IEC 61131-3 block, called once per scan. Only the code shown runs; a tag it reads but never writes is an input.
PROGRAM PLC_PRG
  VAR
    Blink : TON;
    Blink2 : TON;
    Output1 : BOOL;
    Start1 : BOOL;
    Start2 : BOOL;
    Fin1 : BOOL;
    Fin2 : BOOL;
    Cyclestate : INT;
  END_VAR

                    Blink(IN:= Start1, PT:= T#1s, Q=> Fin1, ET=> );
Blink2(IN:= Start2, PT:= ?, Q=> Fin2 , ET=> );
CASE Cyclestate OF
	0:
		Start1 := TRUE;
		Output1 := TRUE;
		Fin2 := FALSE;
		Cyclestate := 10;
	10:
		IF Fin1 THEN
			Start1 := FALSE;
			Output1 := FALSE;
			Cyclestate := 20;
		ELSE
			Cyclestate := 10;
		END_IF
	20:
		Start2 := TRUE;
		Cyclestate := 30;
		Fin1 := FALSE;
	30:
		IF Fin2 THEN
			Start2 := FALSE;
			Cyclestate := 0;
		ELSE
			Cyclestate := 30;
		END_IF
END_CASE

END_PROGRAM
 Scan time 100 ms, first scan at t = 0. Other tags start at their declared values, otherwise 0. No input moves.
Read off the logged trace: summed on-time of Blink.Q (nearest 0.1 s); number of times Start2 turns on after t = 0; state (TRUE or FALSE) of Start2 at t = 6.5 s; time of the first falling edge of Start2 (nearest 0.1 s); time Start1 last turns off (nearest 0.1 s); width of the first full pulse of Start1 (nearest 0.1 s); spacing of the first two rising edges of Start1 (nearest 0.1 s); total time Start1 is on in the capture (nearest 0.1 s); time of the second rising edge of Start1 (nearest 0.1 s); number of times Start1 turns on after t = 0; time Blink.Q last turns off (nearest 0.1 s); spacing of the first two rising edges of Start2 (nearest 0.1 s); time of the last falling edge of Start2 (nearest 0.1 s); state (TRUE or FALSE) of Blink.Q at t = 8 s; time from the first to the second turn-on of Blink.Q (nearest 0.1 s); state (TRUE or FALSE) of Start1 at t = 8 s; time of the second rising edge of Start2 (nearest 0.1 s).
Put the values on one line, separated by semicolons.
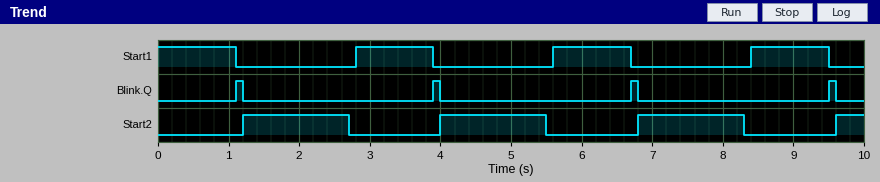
0.4 s; 4; FALSE; 2.7 s; 9.5 s; 1.1 s; 2.8 s; 4.4 s; 5.6 s; 3; 9.6 s; 2.8 s; 8.3 s; FALSE; 2.8 s; FALSE; 4.0 s
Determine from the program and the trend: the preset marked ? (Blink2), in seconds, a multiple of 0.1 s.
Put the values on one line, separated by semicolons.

1.4 s
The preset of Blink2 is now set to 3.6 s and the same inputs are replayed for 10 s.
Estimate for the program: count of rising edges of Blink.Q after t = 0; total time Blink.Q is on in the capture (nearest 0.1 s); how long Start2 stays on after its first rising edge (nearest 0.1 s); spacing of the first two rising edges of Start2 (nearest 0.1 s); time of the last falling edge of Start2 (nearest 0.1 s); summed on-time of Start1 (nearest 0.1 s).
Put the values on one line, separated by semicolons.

2; 0.2 s; 3.7 s; 5.0 s; 9.9 s; 2.2 s
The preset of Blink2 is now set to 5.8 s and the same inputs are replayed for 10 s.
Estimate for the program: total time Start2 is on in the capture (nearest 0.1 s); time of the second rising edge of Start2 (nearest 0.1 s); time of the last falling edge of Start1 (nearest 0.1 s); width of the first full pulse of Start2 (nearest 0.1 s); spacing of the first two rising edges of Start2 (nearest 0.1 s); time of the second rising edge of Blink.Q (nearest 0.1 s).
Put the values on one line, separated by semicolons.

7.5 s; 8.4 s; 8.3 s; 5.9 s; 7.2 s; 8.3 s
